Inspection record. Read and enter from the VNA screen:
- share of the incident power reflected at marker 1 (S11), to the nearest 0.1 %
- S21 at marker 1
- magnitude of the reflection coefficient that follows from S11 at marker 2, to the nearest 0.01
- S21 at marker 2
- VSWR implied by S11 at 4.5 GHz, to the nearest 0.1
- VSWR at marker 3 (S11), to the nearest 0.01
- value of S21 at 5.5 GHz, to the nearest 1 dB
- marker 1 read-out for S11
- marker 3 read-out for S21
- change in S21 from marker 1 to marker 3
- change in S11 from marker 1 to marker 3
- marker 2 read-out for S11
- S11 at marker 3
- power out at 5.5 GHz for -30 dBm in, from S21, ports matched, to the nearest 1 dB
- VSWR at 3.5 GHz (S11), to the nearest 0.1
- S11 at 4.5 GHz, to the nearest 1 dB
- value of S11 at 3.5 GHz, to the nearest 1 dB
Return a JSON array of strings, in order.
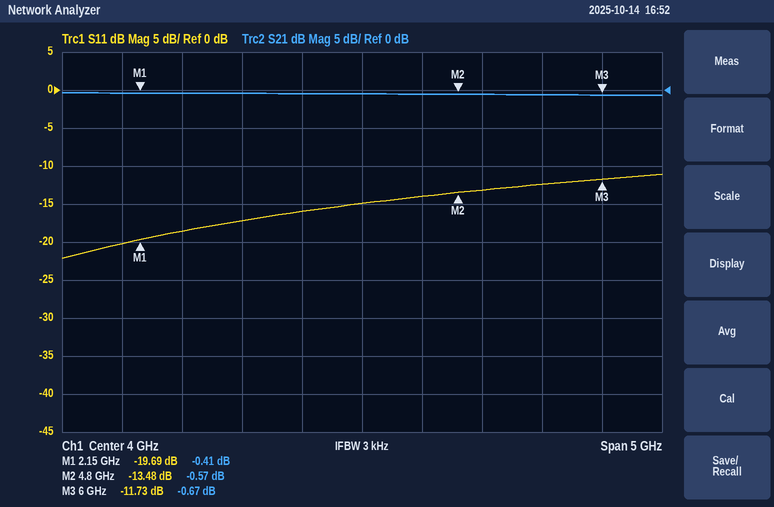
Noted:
["1.1 %", "-0.41 dB", "0.21", "-0.57 dB", "1.5", "1.70", "-1 dB", "-19.69 dB", "-0.67 dB", "-0.26 dB", "7.96 dB", "-13.48 dB", "-11.73 dB", "-31 dBm", "1.4", "-14 dB", "-16 dB"]
